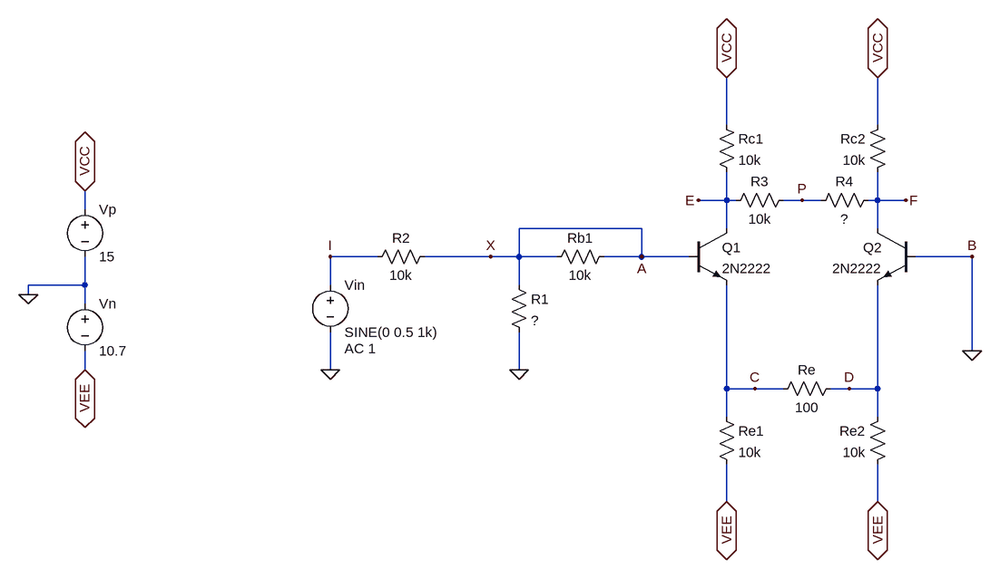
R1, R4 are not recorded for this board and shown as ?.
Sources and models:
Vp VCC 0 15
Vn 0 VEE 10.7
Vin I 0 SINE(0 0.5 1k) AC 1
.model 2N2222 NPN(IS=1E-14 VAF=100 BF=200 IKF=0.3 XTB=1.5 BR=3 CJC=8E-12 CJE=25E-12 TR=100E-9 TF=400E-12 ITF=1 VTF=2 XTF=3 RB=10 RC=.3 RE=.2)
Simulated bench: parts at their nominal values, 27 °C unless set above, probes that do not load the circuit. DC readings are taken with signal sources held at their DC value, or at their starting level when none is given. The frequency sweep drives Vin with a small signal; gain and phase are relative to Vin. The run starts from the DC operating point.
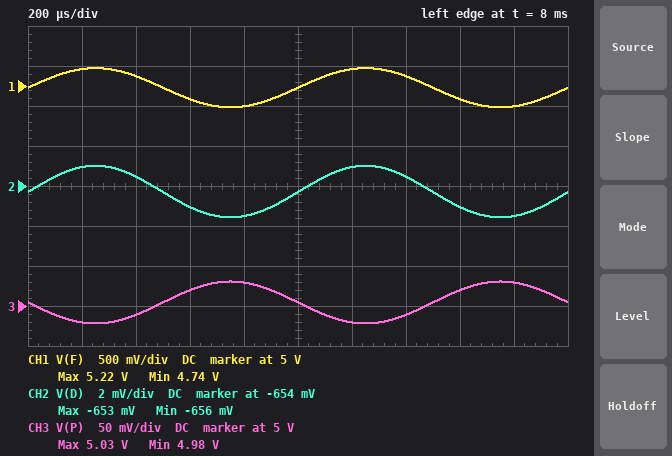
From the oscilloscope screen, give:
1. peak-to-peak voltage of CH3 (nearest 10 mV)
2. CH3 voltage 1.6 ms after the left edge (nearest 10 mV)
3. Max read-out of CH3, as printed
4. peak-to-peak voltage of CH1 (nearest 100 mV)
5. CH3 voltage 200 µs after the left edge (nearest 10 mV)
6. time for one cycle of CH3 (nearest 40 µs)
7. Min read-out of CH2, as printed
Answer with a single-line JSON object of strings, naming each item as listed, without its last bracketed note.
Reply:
{"peak-to-peak voltage of CH3": "50 mV", "CH3 voltage 1.6 ms after the left edge": "5.02 V", "Max read-out of CH3, as printed": "5.03 V", "peak-to-peak voltage of CH1": "500 mV", "CH3 voltage 200 µs after the left edge": "4.98 V", "time for one cycle of CH3": "1.00 ms", "Min read-out of CH2, as printed": "-656 mV"}
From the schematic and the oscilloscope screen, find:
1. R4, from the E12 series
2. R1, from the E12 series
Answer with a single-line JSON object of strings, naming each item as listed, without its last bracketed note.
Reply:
{"R4, from the E12 series": "12 kΩ", "R1, from the E12 series": "150 Ω"}
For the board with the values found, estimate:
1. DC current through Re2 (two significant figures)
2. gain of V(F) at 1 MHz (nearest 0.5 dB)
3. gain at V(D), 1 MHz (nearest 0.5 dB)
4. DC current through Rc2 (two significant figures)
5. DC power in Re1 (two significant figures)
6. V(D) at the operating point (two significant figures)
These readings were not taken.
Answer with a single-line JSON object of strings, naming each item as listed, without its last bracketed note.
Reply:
{"DC current through Re2": "1.0 mA", "gain of V(F) at 1 MHz": "-6.5 dB", "gain at V(D), 1 MHz": "-52.0 dB", "DC current through Rc2": "1.0 mA", "DC power in Re1": "10 mW", "V(D) at the operating point": "-650 mV"}
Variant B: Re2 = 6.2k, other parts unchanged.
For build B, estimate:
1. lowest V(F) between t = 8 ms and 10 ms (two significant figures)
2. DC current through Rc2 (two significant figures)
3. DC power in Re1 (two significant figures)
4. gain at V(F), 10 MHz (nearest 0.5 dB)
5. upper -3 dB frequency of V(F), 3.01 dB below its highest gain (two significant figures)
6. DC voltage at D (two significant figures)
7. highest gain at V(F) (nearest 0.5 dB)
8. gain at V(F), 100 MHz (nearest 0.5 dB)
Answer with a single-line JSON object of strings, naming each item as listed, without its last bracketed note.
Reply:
{"lowest V(F) between t = 8 ms and 10 ms": "540 mV", "DC current through Rc2": "1.4 mA", "DC power in Re1": "10 mW", "gain at V(F), 10 MHz": "-19.0 dB", "upper -3 dB frequency of V(F), 3.01 dB below its highest gain": "2.4 MHz", "DC voltage at D": "-670 mV", "highest gain at V(F)": "-5.5 dB", "gain at V(F), 100 MHz": "-40.0 dB"}
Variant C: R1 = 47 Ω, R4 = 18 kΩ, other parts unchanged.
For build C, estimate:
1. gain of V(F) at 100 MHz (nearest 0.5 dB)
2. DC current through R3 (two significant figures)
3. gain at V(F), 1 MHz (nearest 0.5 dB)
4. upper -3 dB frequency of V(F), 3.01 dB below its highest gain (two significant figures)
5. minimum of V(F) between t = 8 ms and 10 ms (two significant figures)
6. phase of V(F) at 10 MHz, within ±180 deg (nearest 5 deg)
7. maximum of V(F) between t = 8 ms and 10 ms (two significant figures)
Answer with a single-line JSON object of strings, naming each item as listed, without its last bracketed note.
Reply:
{"gain of V(F) at 100 MHz": "-43.5 dB", "DC current through R3": "600 nA", "gain at V(F), 1 MHz": "-15.5 dB", "upper -3 dB frequency of V(F), 3.01 dB below its highest gain": "4.7 MHz", "minimum of V(F) between t = 8 ms and 10 ms": "4.9 V", "phase of V(F) at 10 MHz, within ±180 deg": "-70 deg", "maximum of V(F) between t = 8 ms and 10 ms": "5.1 V"}
